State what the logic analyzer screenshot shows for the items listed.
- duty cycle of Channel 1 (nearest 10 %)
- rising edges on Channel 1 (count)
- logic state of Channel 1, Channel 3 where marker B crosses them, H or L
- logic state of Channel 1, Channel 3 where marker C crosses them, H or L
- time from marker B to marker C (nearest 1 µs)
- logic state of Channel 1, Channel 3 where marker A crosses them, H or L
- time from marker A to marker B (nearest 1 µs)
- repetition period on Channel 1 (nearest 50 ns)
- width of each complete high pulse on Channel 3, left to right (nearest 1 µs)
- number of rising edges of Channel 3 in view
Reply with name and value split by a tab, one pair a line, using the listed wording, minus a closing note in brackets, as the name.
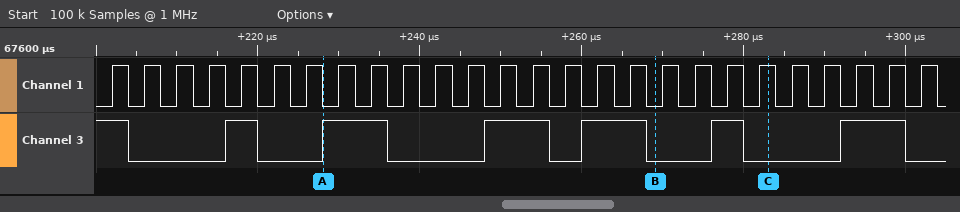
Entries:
duty cycle of Channel 1	50 %
rising edges on Channel 1	26
logic state of Channel 1, Channel 3 where marker B crosses them, H or L	Channel 1=L, Channel 3=L
logic state of Channel 1, Channel 3 where marker C crosses them, H or L	Channel 1=H, Channel 3=L
time from marker B to marker C	14 µs
logic state of Channel 1, Channel 3 where marker A crosses them, H or L	Channel 1=L, Channel 3=H
time from marker A to marker B	41 µs
repetition period on Channel 1	4000 ns
width of each complete high pulse on Channel 3, left to right	4 µs, 8 µs, 8 µs, 8 µs, 4 µs, 8 µs
number of rising edges of Channel 3 in view	6
